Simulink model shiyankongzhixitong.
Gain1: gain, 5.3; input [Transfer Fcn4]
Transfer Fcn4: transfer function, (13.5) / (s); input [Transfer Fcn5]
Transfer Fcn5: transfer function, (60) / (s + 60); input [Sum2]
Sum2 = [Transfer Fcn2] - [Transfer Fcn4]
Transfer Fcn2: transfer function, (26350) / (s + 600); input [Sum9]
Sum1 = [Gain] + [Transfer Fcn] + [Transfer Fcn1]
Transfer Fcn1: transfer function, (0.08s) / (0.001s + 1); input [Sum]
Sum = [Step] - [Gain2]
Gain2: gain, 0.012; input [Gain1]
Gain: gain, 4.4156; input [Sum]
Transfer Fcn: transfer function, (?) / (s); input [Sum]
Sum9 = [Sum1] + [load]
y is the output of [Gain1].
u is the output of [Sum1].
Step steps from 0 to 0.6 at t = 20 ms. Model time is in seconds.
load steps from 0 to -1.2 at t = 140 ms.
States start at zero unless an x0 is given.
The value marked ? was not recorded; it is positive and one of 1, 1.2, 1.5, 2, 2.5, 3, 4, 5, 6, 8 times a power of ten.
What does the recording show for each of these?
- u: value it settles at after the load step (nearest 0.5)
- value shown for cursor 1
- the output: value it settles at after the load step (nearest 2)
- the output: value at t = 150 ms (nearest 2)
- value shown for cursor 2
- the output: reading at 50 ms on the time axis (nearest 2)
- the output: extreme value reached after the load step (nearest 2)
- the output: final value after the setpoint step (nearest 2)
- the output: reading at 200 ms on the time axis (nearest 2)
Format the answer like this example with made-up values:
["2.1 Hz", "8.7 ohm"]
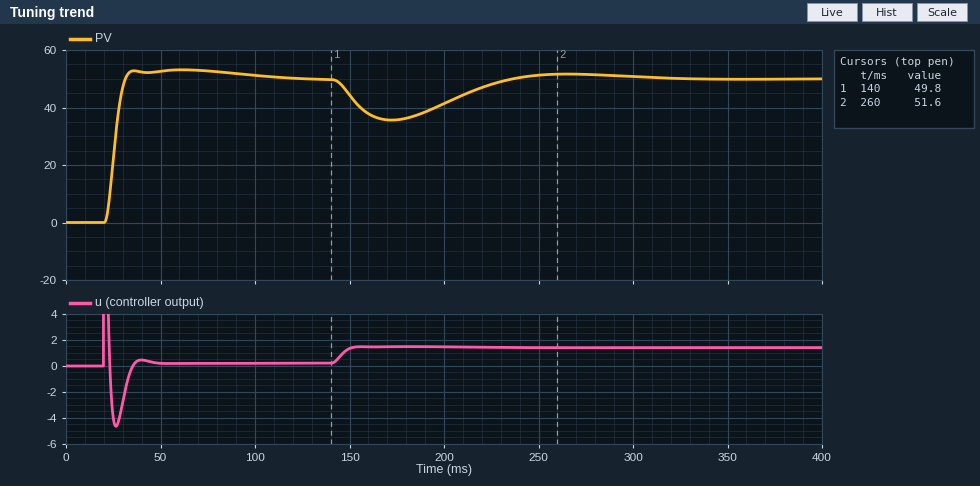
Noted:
["1.5", "49.8", "50", "44", "51.6", "52", "36", "50", "42"]
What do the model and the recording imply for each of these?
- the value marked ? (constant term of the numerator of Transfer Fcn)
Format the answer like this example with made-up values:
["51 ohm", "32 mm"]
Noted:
["150"]
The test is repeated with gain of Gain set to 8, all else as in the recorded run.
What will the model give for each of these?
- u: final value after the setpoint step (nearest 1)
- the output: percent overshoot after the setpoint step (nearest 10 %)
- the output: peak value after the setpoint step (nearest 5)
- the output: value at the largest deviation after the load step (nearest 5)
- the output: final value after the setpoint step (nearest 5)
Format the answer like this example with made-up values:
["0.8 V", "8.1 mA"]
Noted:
["0", "20 %", "60", "40", "50"]
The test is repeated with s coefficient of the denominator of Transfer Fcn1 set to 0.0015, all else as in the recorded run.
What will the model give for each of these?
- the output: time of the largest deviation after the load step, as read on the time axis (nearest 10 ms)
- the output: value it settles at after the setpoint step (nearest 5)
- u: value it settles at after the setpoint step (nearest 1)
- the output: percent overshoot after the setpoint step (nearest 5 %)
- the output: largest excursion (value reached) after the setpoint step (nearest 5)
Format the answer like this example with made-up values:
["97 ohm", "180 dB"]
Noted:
["170 ms", "50", "0", "10 %", "55"]
